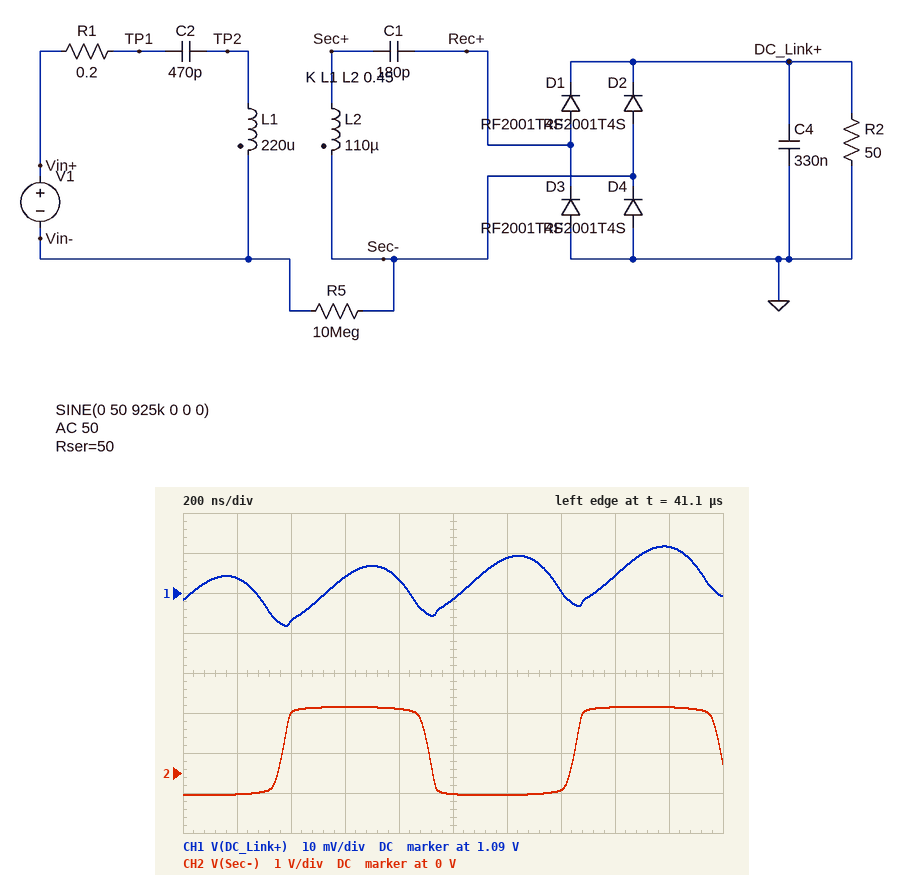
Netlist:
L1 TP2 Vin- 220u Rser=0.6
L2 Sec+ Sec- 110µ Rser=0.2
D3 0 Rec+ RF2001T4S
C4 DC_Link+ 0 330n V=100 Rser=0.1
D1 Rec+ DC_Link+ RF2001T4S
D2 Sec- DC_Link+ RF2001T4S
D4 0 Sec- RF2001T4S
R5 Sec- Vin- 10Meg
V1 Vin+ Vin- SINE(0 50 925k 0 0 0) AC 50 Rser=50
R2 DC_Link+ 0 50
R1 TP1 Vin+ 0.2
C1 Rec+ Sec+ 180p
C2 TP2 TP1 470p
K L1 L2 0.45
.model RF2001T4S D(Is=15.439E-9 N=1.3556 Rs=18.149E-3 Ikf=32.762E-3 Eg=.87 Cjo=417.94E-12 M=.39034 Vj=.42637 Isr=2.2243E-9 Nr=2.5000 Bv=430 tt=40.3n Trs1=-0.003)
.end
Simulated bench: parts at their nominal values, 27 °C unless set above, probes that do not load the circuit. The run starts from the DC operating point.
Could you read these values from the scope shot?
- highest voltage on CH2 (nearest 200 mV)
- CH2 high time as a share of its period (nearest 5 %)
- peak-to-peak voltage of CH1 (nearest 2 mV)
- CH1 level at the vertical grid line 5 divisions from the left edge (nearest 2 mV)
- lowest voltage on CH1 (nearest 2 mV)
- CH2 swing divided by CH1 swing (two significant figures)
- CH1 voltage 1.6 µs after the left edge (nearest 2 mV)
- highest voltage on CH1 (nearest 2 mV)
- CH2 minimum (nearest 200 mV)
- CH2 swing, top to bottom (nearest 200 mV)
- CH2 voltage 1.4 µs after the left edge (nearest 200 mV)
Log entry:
1.6 V
50 %
20 mV
1.088 V
1.082 V
110
1.094 V
1.102 V
-600 mV
2.2 V
-400 mV
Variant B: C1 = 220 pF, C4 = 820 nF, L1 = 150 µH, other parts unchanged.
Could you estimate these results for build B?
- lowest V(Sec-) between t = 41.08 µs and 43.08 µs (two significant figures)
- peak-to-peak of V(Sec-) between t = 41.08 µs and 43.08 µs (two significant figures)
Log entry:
-600 mV
2.9 V
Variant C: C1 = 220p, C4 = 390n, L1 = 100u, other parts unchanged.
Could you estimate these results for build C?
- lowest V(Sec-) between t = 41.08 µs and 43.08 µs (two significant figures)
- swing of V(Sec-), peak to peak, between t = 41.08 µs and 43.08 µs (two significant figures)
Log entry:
-620 mV
4.5 V
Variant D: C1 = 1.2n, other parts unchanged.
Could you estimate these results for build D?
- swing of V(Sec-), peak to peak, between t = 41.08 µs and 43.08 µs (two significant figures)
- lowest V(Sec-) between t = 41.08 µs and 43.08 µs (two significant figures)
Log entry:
3.2 V
-590 mV
